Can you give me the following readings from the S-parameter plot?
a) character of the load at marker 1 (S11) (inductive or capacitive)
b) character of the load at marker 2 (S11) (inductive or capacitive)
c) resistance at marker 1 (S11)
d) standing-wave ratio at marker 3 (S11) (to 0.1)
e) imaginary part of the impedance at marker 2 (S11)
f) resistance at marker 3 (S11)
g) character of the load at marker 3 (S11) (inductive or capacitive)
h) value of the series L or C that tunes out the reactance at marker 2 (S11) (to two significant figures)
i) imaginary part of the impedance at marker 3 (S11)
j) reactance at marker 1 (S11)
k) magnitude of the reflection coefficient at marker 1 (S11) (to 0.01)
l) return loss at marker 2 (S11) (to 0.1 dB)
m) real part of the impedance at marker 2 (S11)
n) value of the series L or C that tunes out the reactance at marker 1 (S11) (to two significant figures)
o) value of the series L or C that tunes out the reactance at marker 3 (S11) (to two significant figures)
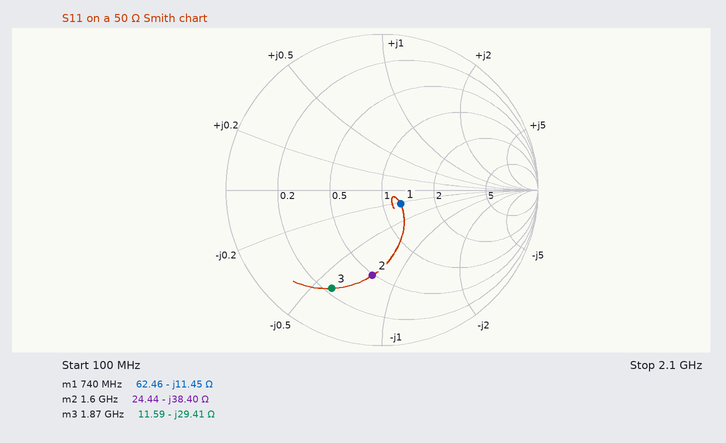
capacitive
capacitive
62.46 Ω
5.9
-38.40 Ω
11.59 Ω
capacitive
3.8 nH
-29.41 Ω
-11.45 Ω
0.15
5.2 dB
24.44 Ω
2.5 nH
2.5 nH
